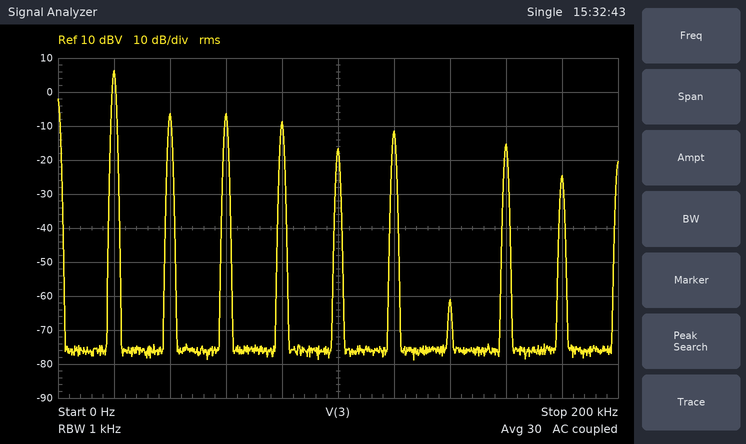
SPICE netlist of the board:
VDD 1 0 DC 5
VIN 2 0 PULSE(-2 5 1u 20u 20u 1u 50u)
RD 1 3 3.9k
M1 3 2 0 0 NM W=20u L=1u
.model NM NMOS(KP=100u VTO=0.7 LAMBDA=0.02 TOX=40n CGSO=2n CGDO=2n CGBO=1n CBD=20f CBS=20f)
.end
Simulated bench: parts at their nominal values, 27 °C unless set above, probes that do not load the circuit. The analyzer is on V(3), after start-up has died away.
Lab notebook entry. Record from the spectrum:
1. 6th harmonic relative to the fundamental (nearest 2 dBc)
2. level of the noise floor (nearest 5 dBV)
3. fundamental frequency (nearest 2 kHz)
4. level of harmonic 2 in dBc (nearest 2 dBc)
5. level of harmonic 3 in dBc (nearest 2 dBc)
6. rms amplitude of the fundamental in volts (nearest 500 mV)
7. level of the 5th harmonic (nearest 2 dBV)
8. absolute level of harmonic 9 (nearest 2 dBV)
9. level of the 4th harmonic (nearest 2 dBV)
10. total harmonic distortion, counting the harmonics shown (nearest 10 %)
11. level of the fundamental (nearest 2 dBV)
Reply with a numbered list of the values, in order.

1. -18 dBc
2. -75 dBV
3. 20 kHz
4. -12 dBc
5. -12 dBc
6. 2.0 V
7. -16 dBV
8. -24 dBV
9. -8 dBV
10. 40 %
11. 6 dBV
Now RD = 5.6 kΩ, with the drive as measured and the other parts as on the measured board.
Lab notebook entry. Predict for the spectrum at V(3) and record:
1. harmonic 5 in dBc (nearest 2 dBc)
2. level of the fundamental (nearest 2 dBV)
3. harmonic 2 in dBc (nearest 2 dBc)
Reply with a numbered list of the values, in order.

1. -20 dBc
2. 6 dBV
3. -14 dBc
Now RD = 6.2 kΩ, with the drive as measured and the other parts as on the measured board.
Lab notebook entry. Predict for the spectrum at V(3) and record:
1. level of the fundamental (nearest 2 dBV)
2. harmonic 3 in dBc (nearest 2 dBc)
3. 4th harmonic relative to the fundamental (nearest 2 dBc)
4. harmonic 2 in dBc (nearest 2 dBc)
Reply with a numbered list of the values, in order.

1. 6 dBV
2. -12 dBc
3. -16 dBc
4. -14 dBc
